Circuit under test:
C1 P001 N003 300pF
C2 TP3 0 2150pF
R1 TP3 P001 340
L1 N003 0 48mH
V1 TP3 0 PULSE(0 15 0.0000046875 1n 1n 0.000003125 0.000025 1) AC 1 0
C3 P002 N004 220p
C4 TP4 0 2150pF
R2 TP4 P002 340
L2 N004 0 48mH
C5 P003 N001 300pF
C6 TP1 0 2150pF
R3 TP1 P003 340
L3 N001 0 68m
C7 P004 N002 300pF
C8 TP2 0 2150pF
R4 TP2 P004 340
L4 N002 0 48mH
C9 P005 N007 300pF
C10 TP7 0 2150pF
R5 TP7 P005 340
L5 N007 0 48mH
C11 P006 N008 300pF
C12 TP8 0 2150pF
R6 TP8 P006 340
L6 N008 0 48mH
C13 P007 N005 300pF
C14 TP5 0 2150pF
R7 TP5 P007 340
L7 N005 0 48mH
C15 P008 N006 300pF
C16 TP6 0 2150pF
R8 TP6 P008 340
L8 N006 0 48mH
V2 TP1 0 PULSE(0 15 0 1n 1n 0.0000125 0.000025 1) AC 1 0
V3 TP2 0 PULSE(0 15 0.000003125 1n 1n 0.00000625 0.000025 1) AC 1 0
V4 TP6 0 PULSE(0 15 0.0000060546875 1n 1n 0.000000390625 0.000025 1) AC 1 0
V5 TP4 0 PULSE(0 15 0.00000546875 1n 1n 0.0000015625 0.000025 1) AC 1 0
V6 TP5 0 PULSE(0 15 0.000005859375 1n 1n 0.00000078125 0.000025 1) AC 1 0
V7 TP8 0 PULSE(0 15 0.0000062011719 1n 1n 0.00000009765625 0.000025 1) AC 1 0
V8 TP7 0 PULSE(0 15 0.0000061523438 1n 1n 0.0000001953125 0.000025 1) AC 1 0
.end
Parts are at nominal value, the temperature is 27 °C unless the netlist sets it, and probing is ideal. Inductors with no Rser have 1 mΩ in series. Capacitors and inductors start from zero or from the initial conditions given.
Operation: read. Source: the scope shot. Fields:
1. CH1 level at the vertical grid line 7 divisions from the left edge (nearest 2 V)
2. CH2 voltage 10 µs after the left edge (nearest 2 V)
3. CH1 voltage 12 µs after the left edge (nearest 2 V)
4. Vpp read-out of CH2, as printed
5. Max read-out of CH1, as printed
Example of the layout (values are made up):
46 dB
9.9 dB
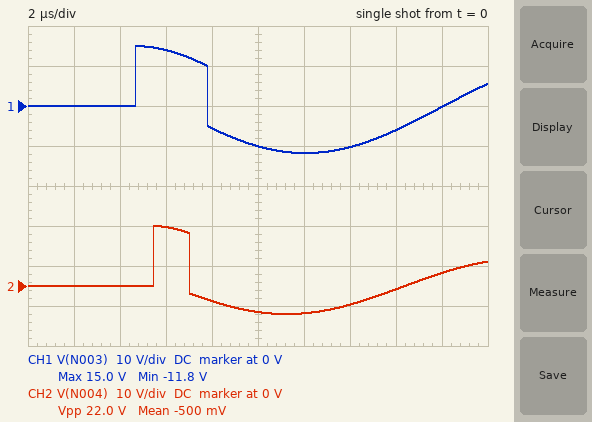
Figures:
-10 V
-6 V
-12 V
22.0 V
15.0 V
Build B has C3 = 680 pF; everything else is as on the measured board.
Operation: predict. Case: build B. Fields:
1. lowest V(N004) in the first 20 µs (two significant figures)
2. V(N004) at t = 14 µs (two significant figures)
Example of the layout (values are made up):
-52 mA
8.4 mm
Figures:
-4.0 V
-3.9 V
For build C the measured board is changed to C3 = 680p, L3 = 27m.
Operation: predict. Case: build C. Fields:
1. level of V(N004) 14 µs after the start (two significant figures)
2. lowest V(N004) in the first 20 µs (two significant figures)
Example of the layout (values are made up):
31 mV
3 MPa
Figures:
-3.9 V
-4.0 V
